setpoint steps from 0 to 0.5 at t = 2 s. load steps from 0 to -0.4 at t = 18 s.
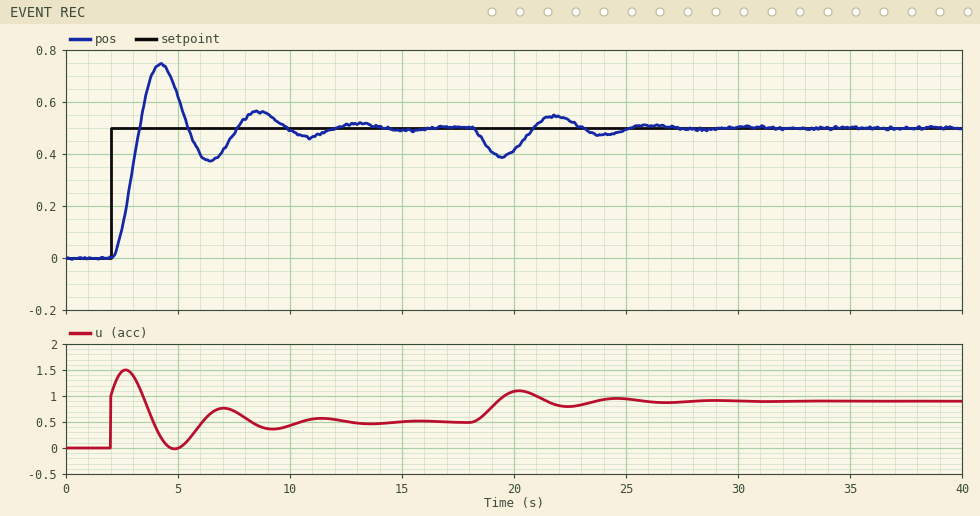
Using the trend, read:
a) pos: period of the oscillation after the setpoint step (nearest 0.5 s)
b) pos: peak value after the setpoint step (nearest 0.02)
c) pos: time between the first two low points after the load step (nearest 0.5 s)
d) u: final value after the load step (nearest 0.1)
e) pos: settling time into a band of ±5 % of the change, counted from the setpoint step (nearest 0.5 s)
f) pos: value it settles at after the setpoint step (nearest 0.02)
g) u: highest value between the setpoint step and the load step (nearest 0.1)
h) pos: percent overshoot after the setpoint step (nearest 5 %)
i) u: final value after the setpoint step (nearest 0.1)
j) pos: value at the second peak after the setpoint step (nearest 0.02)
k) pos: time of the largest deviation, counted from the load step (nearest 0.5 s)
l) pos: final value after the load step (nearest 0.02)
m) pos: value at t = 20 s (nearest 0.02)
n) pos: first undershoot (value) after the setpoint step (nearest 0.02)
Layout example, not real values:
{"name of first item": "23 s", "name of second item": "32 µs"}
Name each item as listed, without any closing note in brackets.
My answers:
{"pos: period of the oscillation after the setpoint step": "4.5 s", "pos: peak value after the setpoint step": "0.74", "pos: time between the first two low points after the load step": "4.5 s", "u: final value after the load step": "0.9", "pos: settling time into a band of ±5 % of the change, counted from the setpoint step": "9.5 s", "pos: value it settles at after the setpoint step": "0.50", "u: highest value between the setpoint step and the load step": "1.5", "pos: percent overshoot after the setpoint step": "50 %", "u: final value after the setpoint step": "0.5", "pos: value at the second peak after the setpoint step": "0.56", "pos: time of the largest deviation, counted from the load step": "1.5 s", "pos: final value after the load step": "0.50", "pos: value at t = 20 s": "0.42", "pos: first undershoot (value) after the setpoint step": "0.38"}
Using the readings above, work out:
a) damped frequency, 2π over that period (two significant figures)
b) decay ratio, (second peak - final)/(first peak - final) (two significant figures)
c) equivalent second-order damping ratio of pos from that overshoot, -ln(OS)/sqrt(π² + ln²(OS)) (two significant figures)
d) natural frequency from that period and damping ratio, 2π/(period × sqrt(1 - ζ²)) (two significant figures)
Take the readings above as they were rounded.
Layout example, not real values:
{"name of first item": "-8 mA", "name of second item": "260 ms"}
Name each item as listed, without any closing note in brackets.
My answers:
{"damped frequency, 2π over that period": "1.4 rad/s", "decay ratio, (second peak - final)/(first peak - final)": "0.25", "equivalent second-order damping ratio of pos from that overshoot, -ln(OS)/sqrt(π² + ln²(OS))": "0.22", "natural frequency from that period and damping ratio, 2π/(period × sqrt(1 - ζ²))": "1.4 rad/s"}
